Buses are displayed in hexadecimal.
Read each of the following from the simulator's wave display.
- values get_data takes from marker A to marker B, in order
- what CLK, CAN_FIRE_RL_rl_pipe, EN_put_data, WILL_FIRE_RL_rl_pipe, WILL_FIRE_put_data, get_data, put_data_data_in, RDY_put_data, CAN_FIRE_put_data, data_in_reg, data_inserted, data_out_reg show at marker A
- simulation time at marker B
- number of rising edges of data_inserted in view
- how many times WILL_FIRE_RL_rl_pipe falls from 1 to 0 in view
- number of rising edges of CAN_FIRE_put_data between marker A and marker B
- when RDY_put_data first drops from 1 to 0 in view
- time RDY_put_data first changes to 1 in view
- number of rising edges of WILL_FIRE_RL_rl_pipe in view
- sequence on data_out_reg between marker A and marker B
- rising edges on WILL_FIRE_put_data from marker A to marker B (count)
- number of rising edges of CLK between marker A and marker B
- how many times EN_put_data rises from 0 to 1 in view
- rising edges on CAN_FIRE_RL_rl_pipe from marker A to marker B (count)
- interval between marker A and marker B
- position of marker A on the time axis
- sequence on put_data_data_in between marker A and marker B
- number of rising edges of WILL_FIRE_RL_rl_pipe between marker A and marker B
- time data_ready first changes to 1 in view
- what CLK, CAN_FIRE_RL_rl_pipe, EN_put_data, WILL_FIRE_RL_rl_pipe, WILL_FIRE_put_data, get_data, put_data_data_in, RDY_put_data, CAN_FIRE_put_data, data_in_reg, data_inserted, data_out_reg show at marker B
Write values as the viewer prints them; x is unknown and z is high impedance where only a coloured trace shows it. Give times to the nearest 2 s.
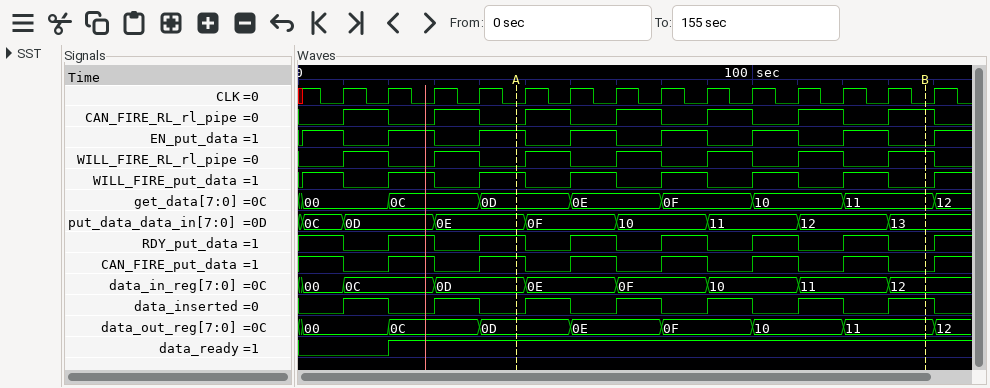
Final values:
0D, 0E, 0F, 10, 11
CLK=0, CAN_FIRE_RL_rl_pipe=0, EN_put_data=1, WILL_FIRE_RL_rl_pipe=0, WILL_FIRE_put_data=1, get_data=0D, put_data_data_in=0E, RDY_put_data=1, CAN_FIRE_put_data=1, data_in_reg=0D, data_inserted=0, data_out_reg=0D
138 s
7
7
4
10 s
20 s
7
0D, 0E, 0F, 10, 11
4
9
8
5
90 s
48 s
0E, 0F, 10, 11, 12, 13
5
20 s
CLK=0, CAN_FIRE_RL_rl_pipe=1, EN_put_data=0, WILL_FIRE_RL_rl_pipe=1, WILL_FIRE_put_data=0, get_data=11, put_data_data_in=13, RDY_put_data=0, CAN_FIRE_put_data=0, data_in_reg=12, data_inserted=1, data_out_reg=11
